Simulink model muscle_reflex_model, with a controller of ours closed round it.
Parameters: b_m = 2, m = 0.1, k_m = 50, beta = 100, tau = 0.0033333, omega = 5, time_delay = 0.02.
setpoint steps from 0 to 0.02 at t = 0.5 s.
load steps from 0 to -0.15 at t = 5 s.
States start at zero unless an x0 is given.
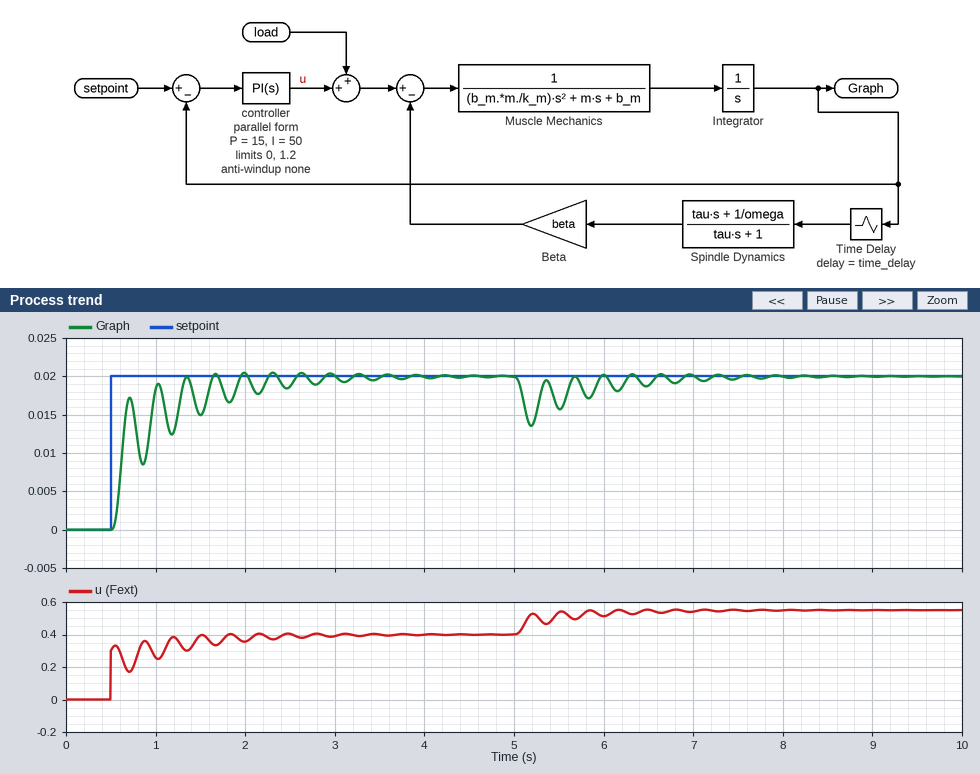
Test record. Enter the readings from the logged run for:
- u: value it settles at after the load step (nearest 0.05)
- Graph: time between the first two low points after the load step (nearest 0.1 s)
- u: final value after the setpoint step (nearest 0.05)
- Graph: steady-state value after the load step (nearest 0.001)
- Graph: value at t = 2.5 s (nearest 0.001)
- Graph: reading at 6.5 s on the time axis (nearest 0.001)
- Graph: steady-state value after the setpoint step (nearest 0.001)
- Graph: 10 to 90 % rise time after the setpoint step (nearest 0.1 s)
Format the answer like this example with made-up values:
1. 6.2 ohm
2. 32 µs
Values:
1. 0.55
2. 0.3 s
3. 0.40
4. 0.020
5. 0.019
6. 0.019
7. 0.020
8. 0.4 s
